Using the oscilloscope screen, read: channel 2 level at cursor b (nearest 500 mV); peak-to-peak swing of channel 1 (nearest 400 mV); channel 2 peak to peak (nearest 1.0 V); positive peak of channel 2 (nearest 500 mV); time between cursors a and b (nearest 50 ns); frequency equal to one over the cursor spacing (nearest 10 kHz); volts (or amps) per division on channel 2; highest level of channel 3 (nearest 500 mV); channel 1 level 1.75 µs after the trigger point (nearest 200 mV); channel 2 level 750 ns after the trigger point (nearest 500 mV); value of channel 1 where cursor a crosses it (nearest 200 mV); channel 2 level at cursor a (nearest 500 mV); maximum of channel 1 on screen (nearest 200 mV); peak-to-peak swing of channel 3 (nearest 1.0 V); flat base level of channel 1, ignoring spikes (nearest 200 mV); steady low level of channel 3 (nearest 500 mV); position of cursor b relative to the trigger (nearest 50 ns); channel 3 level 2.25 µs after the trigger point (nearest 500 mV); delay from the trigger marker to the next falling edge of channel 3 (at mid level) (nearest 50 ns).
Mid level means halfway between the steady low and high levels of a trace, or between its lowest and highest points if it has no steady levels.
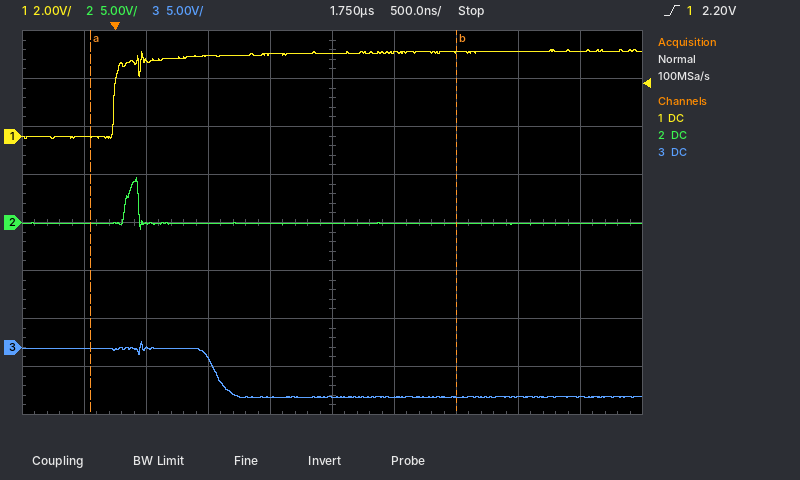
0.0 V
3.6 V
5.0 V
4.5 V
2.95 µs
340 kHz
5 V
500 mV
3.4 V
0.0 V
0.0 V
0.0 V
3.6 V
6.0 V
0.0 V
-5.0 V
+2.75 µs
-5.0 V
800 ns
